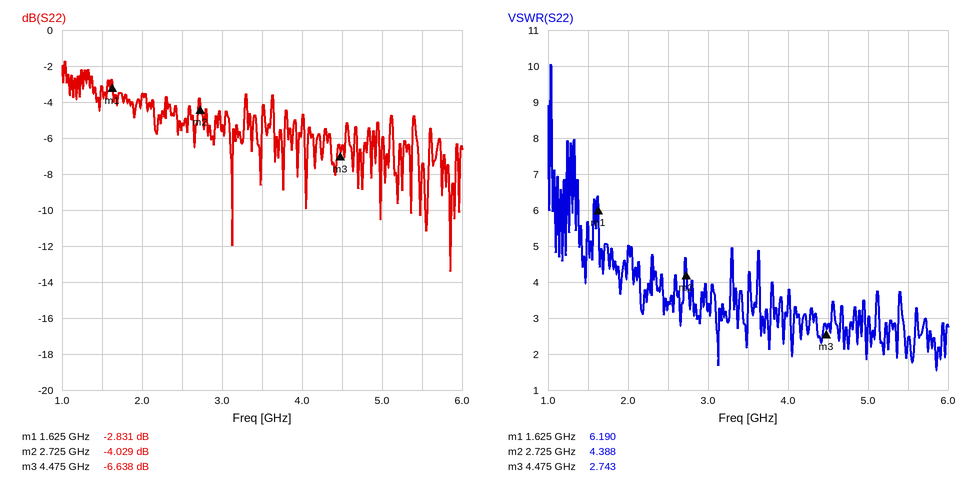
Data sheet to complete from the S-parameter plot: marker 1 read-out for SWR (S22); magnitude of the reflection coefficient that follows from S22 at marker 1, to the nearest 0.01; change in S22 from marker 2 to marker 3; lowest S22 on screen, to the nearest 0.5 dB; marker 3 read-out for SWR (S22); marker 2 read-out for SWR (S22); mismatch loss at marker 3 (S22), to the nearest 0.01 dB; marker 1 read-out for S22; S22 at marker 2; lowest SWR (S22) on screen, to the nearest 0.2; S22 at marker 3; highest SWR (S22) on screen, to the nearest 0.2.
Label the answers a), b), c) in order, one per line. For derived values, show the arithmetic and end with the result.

a) 6.190
b) 10^(-2.831/20) ≈ 0.72
c) -6.638 − (-4.029) = -2.609 dB
d) -13.5 dB
e) 2.743
f) 4.388
g) −10 log10(1 − 10^(-6.638/10)) ≈ 1.06 dB
h) -2.831 dB
i) -4.029 dB
j) 1.6
k) -6.638 dB
l) 10.0
